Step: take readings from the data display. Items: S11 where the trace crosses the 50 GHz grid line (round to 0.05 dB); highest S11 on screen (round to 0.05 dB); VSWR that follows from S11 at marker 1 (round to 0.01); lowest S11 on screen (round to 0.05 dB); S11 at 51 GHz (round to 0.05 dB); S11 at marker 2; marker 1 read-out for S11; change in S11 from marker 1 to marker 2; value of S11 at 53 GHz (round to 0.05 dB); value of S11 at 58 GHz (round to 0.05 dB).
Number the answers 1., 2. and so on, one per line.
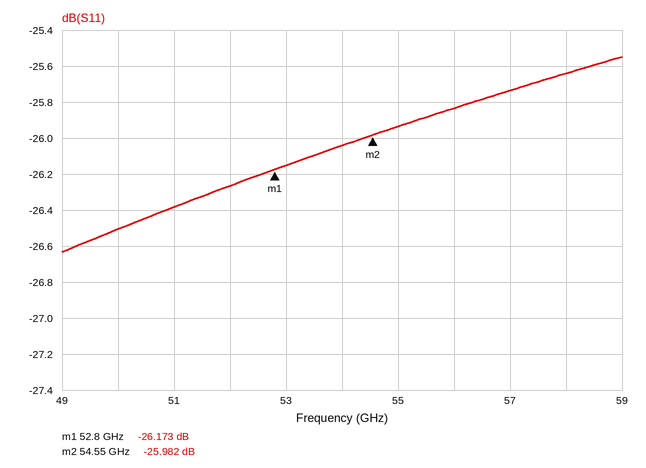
1. -26.50 dB
2. -25.55 dB
3. 1.10
4. -26.65 dB
5. -26.40 dB
6. -25.982 dB
7. -26.173 dB
8. 0.191 dB
9. -26.15 dB
10. -25.65 dB
